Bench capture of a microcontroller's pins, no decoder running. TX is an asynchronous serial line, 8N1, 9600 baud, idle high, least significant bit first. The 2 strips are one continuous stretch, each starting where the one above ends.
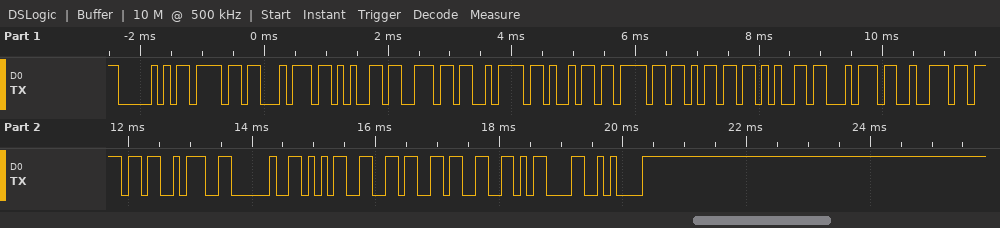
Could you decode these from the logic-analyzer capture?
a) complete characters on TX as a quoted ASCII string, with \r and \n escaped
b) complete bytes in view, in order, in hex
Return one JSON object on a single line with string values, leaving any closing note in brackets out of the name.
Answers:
{"complete characters on TX as a quoted ASCII string, with \\r and \\n escaped": "\"Potenziometro: 563\\r\\n\"", "complete bytes in view, in order, in hex": "50 6F 74 65 6E 7A 69 6F 6D 65 74 72 6F 3A 20 35 36 33 0D 0A"}
